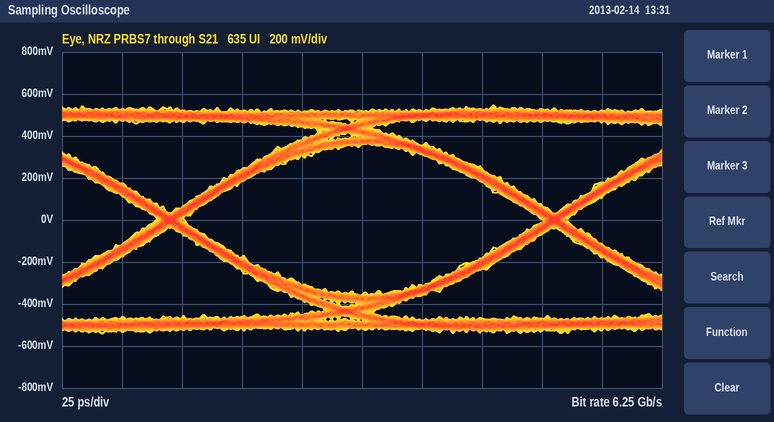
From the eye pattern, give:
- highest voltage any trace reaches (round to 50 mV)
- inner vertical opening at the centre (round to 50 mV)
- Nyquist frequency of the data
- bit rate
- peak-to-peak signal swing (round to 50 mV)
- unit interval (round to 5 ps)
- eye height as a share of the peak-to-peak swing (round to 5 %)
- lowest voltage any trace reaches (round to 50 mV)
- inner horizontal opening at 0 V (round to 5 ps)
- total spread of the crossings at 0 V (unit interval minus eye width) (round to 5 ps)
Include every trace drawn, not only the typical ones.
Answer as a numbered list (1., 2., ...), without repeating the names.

1. 550 mV
2. 700 mV
3. 3.125 GHz
4. 6.25 Gb/s
5. 1.10 V
6. 160 ps
7. 65 %
8. -550 mV
9. 150 ps
10. 10 ps
